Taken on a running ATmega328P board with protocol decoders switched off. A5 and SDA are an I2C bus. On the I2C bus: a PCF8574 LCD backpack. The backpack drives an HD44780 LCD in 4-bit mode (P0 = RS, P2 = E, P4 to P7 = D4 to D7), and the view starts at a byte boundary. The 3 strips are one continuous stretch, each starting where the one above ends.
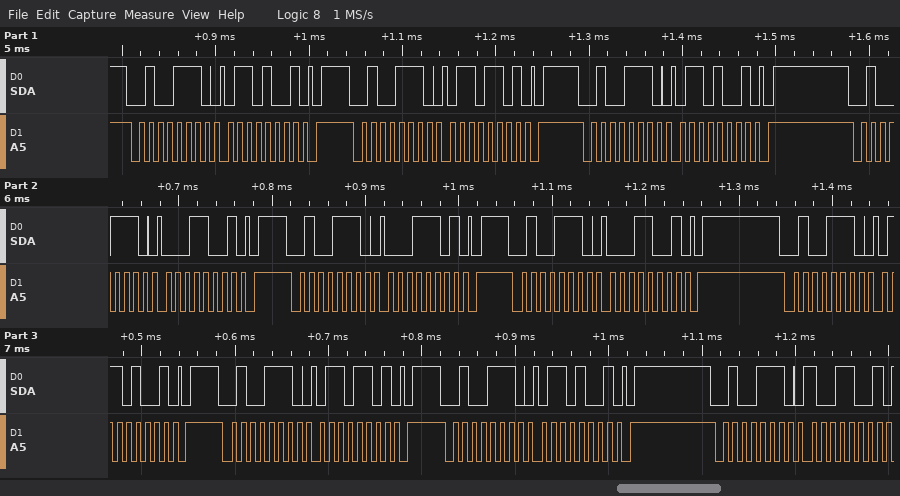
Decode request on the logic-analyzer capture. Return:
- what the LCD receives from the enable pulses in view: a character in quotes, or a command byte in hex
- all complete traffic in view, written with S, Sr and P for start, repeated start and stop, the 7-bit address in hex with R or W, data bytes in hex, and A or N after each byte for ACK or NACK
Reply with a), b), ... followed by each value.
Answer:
a) 'a'
b) S 27W A 69 A P S 27W A 6D A P S 27W A 69 A P S 27W A 19 A P S 27W A 1D A P S 27W A 19 A P S 27W A 69 A P S 27W A 6D A P S 27W A 69 A P S 27W A 99 A
